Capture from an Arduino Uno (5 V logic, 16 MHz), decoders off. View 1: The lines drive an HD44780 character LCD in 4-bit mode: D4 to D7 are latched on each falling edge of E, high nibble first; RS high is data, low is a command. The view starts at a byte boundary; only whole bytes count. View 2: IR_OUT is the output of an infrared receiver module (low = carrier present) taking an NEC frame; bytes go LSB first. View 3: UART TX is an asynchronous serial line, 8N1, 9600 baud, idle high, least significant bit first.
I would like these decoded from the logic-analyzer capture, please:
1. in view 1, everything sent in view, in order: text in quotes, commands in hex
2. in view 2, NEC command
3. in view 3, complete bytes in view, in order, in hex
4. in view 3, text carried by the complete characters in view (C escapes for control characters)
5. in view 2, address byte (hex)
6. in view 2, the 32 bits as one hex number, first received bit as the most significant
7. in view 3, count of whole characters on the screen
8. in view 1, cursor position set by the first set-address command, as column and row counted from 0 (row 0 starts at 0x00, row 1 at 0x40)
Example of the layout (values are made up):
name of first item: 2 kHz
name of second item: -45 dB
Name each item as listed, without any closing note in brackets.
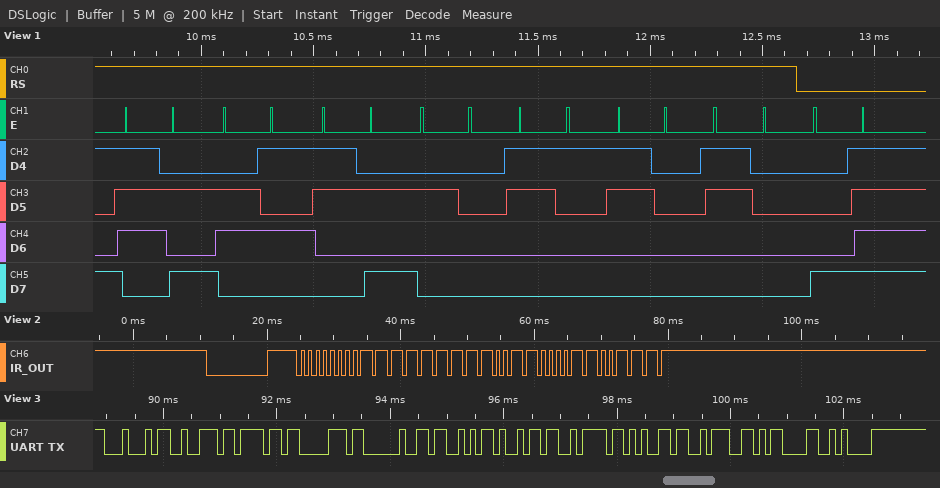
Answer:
in view 1, everything sent in view, in order: text in quotes, commands in hex: "ze: 100" 0x8F
in view 2, NEC command: 0x19
in view 3, complete bytes in view, in order, in hex: 44 72 6F 70 20 53 69 7A 65 3A 0D 0A
in view 3, text carried by the complete characters in view: "Drop Size:\r\n"
in view 2, address byte: 0x00
in view 2, the 32 bits as one hex number, first received bit as the most significant: 0x00FF9867
in view 3, count of whole characters on the screen: 12
in view 1, cursor position set by the first set-address command, as column and row counted from 0: column 15, row 0
